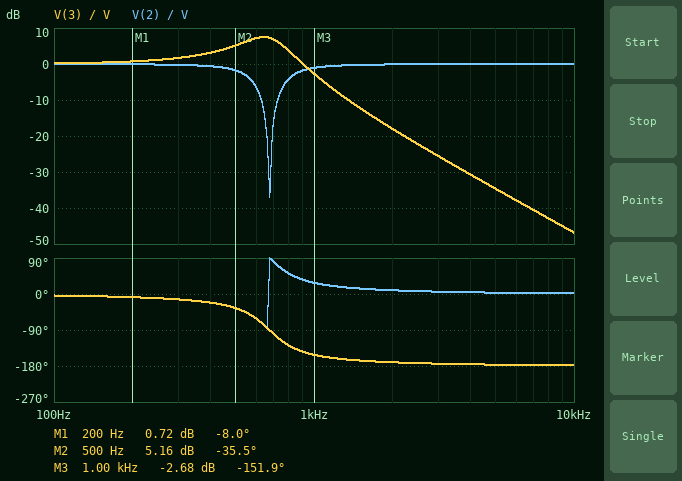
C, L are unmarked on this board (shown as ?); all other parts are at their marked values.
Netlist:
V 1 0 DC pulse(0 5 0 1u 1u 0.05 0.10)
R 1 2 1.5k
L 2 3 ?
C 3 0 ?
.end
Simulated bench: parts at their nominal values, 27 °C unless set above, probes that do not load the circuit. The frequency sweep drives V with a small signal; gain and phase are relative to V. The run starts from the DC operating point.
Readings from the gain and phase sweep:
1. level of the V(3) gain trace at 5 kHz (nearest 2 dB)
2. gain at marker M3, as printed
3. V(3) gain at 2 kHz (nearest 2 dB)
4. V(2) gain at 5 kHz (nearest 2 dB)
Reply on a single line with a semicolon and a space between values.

-34 dB; -2.68 dB; -18 dB; 0 dB
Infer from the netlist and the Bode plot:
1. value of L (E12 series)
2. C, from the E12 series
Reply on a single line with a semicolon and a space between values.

820 mH; 68 nF
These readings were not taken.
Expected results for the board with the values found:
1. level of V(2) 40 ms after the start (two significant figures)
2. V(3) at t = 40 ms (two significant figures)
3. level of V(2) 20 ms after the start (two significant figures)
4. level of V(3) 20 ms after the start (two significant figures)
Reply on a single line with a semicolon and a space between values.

5.0 V; 5.0 V; 5.0 V; 5.0 V
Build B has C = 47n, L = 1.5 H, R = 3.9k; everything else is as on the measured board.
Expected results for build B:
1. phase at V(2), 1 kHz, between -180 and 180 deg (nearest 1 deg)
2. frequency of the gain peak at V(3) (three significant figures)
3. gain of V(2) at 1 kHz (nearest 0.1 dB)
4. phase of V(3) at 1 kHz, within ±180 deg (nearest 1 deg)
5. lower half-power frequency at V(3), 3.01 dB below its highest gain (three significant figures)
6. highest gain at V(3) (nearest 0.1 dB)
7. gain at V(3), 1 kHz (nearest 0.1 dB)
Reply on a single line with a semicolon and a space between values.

33 deg; 523 Hz; -1.5 dB; -147 deg; 202 Hz; 3.8 dB; -6.5 dB
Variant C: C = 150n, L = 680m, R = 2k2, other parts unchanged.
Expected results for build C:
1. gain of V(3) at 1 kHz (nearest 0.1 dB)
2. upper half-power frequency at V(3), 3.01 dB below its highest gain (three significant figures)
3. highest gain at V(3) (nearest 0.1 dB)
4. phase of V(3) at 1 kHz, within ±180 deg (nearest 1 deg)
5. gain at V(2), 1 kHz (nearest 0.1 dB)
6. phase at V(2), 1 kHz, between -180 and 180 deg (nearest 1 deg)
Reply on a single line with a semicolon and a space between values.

-11.3 dB; 579 Hz; 1.1 dB; -146 deg; -1.7 dB; 34 deg
